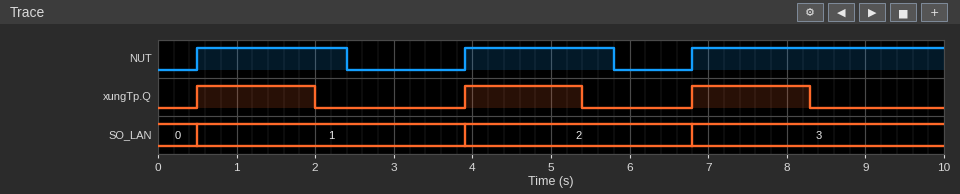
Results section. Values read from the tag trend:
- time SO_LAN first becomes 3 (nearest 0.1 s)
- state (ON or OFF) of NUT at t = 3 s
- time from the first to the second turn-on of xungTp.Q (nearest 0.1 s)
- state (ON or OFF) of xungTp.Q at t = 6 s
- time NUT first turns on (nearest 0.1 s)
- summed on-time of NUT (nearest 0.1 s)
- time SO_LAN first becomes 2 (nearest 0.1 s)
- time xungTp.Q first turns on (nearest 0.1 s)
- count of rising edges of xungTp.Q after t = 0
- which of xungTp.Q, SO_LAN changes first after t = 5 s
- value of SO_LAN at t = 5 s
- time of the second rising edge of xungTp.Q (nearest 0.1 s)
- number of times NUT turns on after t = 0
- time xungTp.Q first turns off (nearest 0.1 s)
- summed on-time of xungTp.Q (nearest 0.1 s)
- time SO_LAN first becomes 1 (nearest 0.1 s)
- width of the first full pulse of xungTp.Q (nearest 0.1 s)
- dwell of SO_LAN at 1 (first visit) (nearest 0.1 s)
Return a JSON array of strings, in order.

["6.8 s", "OFF", "3.4 s", "OFF", "0.5 s", "7.0 s", "3.9 s", "0.5 s", "3", "xungTp.Q", "2", "3.9 s", "3", "2.0 s", "4.5 s", "0.5 s", "1.5 s", "3.4 s"]
